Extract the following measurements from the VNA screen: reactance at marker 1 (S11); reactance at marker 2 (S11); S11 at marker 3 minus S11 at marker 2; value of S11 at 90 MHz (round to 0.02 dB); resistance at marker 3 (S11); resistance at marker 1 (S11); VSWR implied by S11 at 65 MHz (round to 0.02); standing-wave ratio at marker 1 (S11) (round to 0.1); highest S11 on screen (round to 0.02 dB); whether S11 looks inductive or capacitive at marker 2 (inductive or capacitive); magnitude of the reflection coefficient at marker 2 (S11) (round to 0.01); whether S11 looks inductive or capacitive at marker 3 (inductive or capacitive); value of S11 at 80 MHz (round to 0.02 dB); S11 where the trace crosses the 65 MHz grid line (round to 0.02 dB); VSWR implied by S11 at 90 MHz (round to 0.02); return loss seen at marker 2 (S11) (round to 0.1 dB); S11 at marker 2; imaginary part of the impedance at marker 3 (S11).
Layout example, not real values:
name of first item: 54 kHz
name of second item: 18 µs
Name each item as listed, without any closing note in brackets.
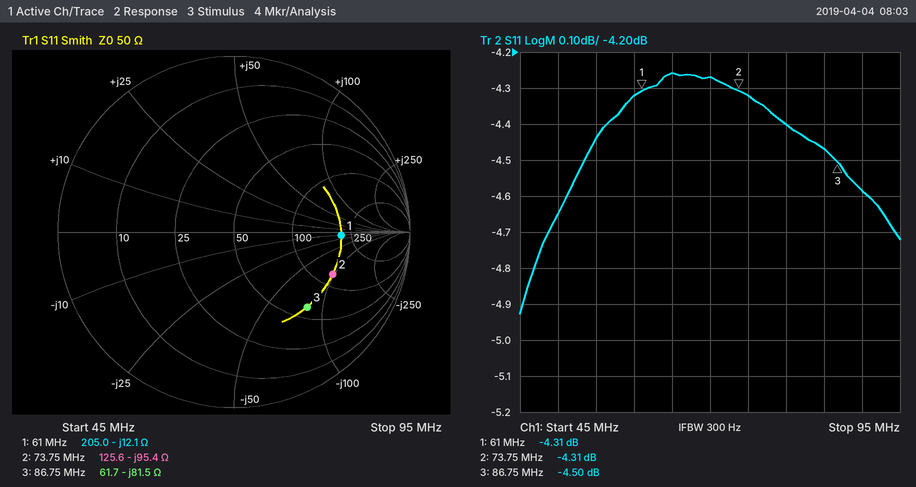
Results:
reactance at marker 1: -12.1 Ω
reactance at marker 2: -95.4 Ω
S11 at marker 3 minus S11 at marker 2: -0.19 dB
value of S11 at 90 MHz: -4.58 dB
resistance at marker 3: 61.7 Ω
resistance at marker 1: 205.0 Ω
VSWR implied by S11 at 65 MHz: 4.16
standing-wave ratio at marker 1 (S11): 4.1
highest S11 on screen: -4.26 dB
whether S11 looks inductive or capacitive at marker 2: capacitive
magnitude of the reflection coefficient at marker 2 (S11): 0.61
whether S11 looks inductive or capacitive at marker 3: capacitive
value of S11 at 80 MHz: -4.40 dB
S11 where the trace crosses the 65 MHz grid line: -4.26 dB
VSWR implied by S11 at 90 MHz: 3.88
return loss seen at marker 2 (S11): 4.3 dB
S11 at marker 2: -4.31 dB
imaginary part of the impedance at marker 3: -81.5 Ω
